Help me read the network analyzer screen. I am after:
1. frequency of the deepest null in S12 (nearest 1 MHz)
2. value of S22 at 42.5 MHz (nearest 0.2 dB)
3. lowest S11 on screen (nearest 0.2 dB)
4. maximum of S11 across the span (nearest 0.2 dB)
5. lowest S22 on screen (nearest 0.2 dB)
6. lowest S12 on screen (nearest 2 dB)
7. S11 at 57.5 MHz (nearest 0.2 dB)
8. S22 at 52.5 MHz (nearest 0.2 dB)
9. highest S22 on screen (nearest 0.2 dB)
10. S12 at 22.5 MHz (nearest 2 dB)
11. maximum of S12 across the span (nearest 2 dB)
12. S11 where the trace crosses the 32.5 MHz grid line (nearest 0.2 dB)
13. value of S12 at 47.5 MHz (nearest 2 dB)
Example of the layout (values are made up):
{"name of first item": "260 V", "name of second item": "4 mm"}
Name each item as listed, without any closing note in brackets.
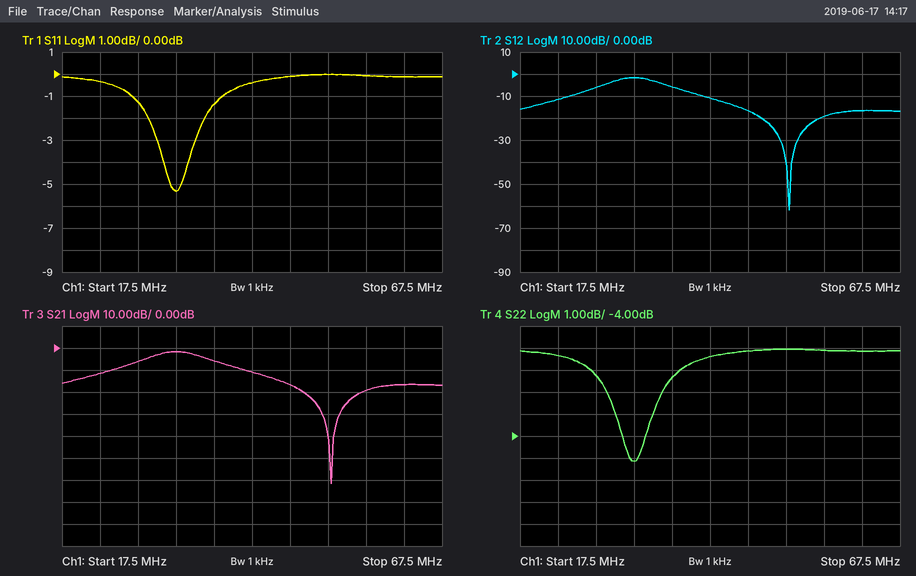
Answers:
{"frequency of the deepest null in S12": "53 MHz", "value of S22 at 42.5 MHz": "-0.4 dB", "lowest S11 on screen": "-5.4 dB", "maximum of S11 across the span": "0.0 dB", "lowest S22 on screen": "-5.2 dB", "lowest S12 on screen": "-62 dB", "S11 at 57.5 MHz": "0.0 dB", "S22 at 52.5 MHz": "0.0 dB", "highest S22 on screen": "0.0 dB", "S12 at 22.5 MHz": "-12 dB", "maximum of S12 across the span": "-2 dB", "S11 where the trace crosses the 32.5 MHz grid line": "-5.4 dB", "value of S12 at 47.5 MHz": "-16 dB"}
